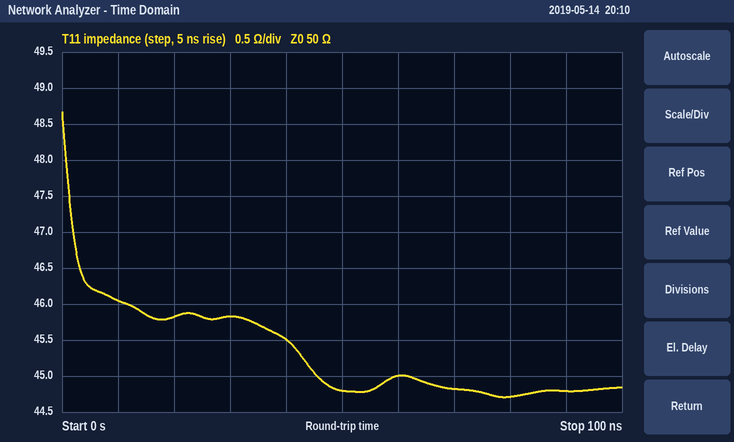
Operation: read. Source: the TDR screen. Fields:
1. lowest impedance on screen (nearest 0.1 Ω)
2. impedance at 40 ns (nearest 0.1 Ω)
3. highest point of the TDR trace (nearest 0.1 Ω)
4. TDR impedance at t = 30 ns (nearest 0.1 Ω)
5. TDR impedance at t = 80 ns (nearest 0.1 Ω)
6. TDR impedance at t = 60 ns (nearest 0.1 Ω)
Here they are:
44.7 Ω
45.5 Ω
48.7 Ω
45.8 Ω
44.7 Ω
45.0 Ω
